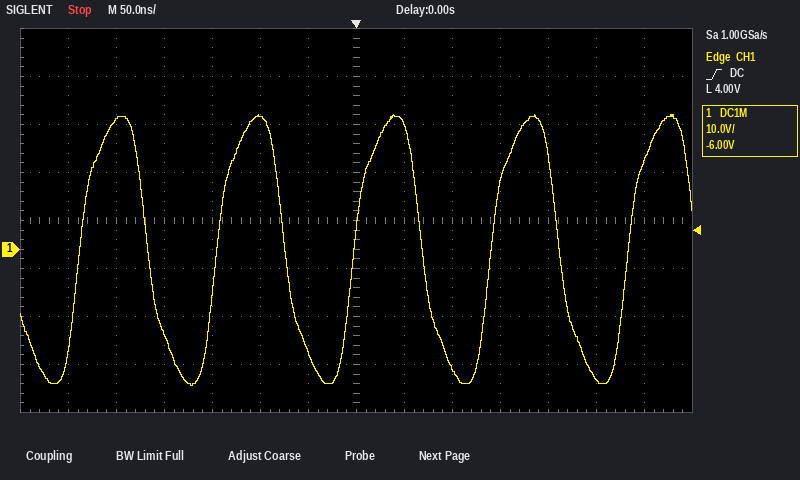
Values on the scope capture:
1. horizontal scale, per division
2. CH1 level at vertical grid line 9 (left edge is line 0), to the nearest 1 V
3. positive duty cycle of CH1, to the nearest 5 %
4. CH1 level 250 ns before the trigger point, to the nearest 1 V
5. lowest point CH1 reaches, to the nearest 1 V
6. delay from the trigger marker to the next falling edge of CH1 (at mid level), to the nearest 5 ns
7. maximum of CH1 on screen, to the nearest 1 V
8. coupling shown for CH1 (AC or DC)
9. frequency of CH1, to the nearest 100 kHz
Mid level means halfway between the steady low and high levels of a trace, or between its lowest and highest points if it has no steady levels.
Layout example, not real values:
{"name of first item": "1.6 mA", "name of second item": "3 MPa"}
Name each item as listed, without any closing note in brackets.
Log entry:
{"horizontal scale, per division": "50 ns", "CH1 level at vertical grid line 9 (left edge is line 0), to the nearest 1 V": "-25 V", "positive duty cycle of CH1, to the nearest 5 %": "50 %", "CH1 level 250 ns before the trigger point, to the nearest 1 V": "27 V", "lowest point CH1 reaches, to the nearest 1 V": "-28 V", "delay from the trigger marker to the next falling edge of CH1 (at mid level), to the nearest 5 ns": "70 ns", "maximum of CH1 on screen, to the nearest 1 V": "28 V", "coupling shown for CH1": "DC", "frequency of CH1, to the nearest 100 kHz": "7.0 MHz"}
